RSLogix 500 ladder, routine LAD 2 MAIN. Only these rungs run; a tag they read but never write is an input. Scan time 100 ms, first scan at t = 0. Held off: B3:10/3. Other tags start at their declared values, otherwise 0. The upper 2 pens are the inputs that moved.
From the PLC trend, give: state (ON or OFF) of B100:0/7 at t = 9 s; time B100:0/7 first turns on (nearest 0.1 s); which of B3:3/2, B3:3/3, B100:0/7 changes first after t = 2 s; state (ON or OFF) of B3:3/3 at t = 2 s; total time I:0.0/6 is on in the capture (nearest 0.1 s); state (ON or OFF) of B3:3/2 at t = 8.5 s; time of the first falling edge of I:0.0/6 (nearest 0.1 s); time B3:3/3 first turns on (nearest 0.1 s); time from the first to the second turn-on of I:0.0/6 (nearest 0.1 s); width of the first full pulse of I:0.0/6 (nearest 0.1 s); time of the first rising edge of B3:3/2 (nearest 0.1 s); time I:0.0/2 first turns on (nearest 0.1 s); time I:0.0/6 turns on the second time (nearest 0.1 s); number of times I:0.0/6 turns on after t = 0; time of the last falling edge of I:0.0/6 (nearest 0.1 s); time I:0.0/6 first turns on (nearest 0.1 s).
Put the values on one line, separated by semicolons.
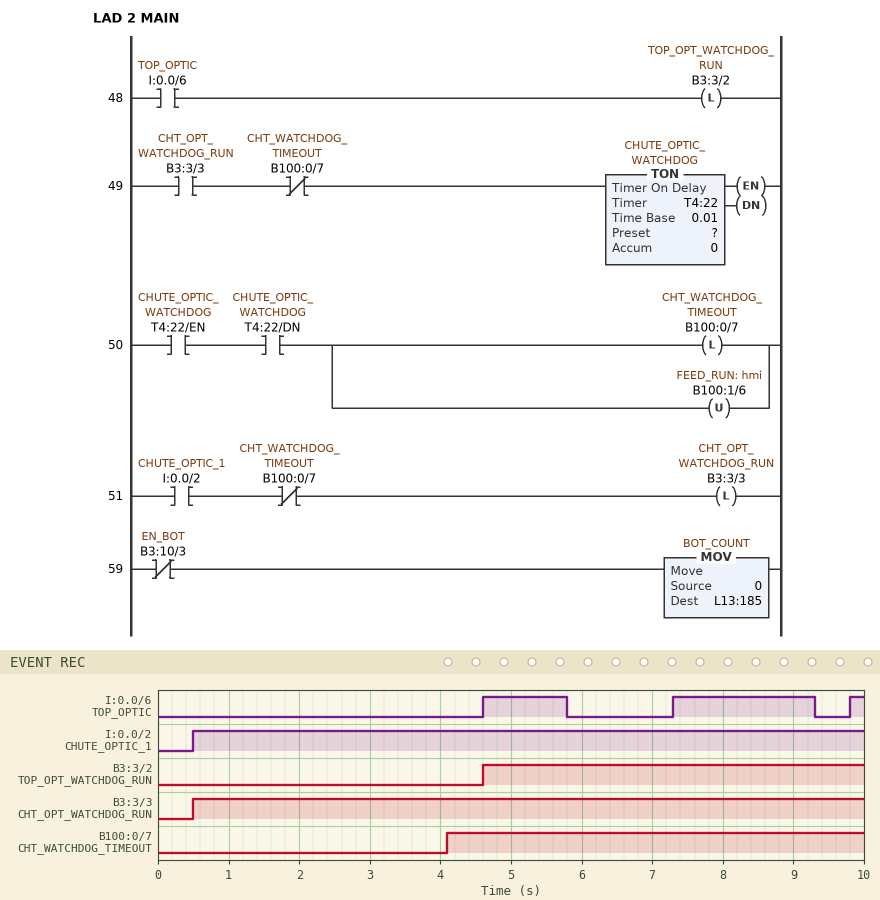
ON; 4.1 s; B100:0/7; ON; 3.4 s; ON; 5.8 s; 0.5 s; 2.7 s; 1.2 s; 4.6 s; 0.5 s; 7.3 s; 3; 9.3 s; 4.6 s
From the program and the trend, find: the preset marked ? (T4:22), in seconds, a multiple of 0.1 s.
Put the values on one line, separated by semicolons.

3.5 s
